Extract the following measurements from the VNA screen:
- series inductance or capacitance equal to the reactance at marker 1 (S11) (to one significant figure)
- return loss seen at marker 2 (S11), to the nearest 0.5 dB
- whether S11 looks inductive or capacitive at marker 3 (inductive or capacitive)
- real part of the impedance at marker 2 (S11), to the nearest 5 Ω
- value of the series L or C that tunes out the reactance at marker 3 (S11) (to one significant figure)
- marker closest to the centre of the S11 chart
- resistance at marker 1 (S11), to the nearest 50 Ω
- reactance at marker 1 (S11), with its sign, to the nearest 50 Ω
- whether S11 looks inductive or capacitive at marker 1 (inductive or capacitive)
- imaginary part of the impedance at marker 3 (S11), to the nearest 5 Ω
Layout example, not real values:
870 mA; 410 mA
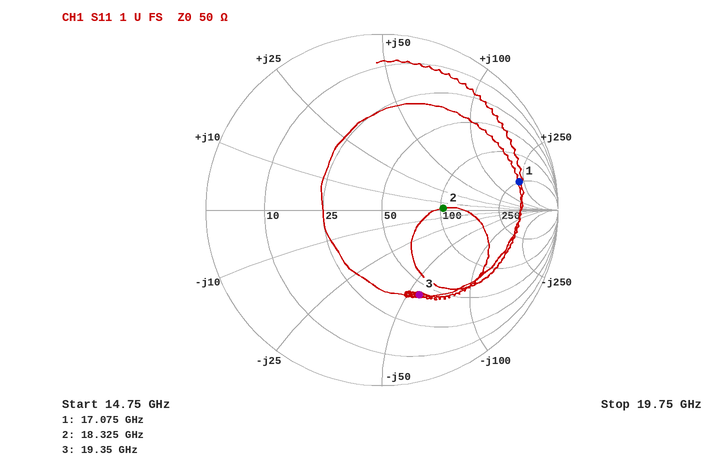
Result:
2 nH; 9.0 dB; capacitive; 105 Ω; 500 pH; marker 2; 250 Ω; +200 Ω; inductive; -55 Ω
